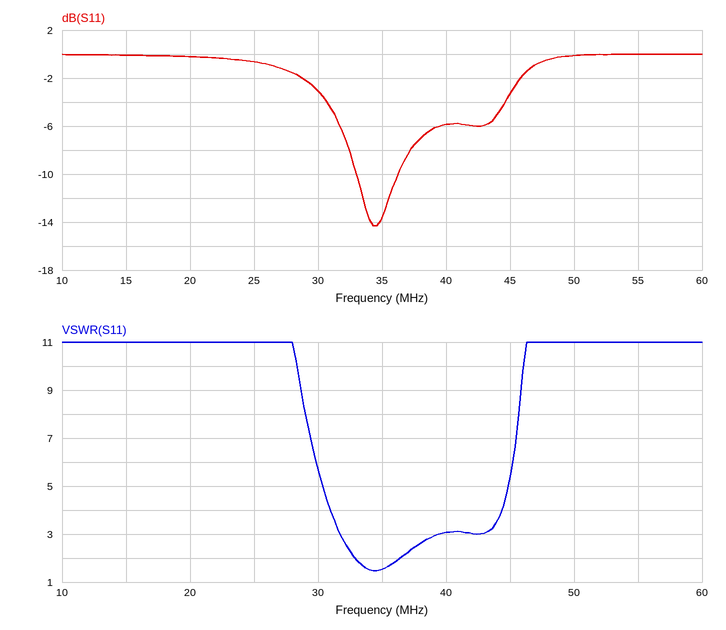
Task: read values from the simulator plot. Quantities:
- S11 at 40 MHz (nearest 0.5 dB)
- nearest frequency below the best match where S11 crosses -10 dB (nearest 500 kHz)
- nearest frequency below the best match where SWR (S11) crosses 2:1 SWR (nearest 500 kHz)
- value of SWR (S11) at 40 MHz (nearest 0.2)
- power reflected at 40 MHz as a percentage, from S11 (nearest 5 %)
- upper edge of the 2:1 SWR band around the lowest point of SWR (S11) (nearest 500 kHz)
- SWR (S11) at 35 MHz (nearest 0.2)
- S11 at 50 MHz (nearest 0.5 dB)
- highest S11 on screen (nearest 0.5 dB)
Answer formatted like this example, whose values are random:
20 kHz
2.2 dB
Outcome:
-6.0 dB
33.0 MHz
33.0 MHz
3.0
25 %
36.5 MHz
1.6
0.0 dB
0.0 dB
